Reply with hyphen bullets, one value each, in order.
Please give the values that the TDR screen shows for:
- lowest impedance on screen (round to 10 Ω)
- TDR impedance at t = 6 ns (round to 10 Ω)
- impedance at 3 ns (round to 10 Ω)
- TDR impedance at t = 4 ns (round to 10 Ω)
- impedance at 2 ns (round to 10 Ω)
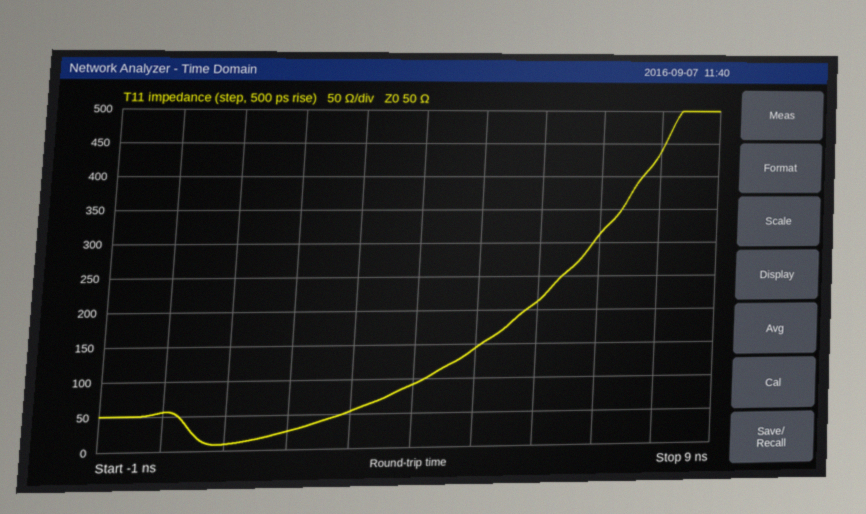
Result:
- 10 Ω
- 210 Ω
- 50 Ω
- 90 Ω
- 30 Ω
